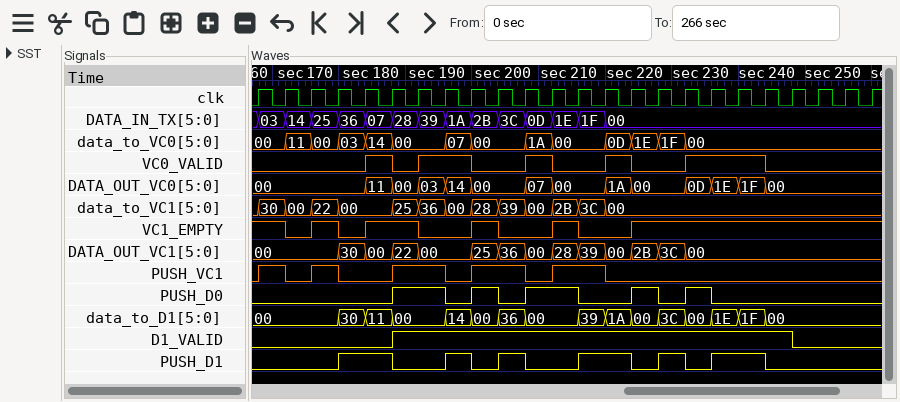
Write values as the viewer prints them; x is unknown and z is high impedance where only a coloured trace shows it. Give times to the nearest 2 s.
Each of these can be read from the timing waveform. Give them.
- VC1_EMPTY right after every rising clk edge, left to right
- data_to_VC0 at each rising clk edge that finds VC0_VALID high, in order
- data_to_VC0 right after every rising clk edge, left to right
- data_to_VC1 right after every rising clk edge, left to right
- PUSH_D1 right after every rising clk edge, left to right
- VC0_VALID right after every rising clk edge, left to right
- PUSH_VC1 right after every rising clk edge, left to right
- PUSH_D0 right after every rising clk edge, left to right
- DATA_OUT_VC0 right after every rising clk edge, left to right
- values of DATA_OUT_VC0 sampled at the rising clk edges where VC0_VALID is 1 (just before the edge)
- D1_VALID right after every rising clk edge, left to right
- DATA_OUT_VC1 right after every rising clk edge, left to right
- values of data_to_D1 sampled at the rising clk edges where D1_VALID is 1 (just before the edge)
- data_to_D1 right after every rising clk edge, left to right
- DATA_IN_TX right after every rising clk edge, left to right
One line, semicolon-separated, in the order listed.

1 0 1 0 1 1 0 0 1 0 0 1 0 0 1 1 1 1 1 1 1 1 1 1; 14, 00, 07, 1A, 0D, 00, 00, 00; 00, 11, 00, 03, 14, 00, 00, 07, 00, 00, 1A, 00, 00, 0D, 1E, 1F, 00, 00, 00, 00, 00, 00, 00, 00; 30, 00, 22, 00, 00, 25, 36, 00, 28, 39, 00, 2B, 3C, 00, 00, 00, 00, 00, 00, 00, 00, 00, 00, 00; 0 0 0 1 1 0 0 1 0 1 0 0 1 1 0 1 0 1 1 0 0 0 0 0; 0 0 0 0 1 0 1 1 0 0 1 0 0 1 0 0 1 1 1 0 0 0 0 0; 1 0 1 0 0 1 1 0 1 1 0 1 1 0 0 0 0 0 0 0 0 0 0 0; 0 0 0 0 0 1 1 0 1 0 1 1 0 0 1 0 1 0 0 0 0 0 0 0; 00, 00, 00, 00, 11, 00, 03, 14, 00, 00, 07, 00, 00, 1A, 00, 00, 0D, 1E, 1F, 00, 00, 00, 00, 00; 11, 03, 14, 07, 1A, 0D, 1E, 1F; 0 0 0 0 0 1 1 1 1 1 1 1 1 1 1 1 1 1 1 1 0 0 0 0; 00, 00, 00, 30, 00, 22, 00, 00, 25, 36, 00, 28, 39, 00, 2B, 3C, 00, 00, 00, 00, 00, 00, 00, 00; 00, 00, 14, 00, 36, 00, 00, 39, 1A, 00, 3C, 00, 1E, 1F, 00; 00, 00, 00, 30, 11, 00, 00, 14, 00, 36, 00, 00, 39, 1A, 00, 3C, 00, 1E, 1F, 00, 00, 00, 00, 00; 03, 14, 25, 36, 07, 28, 39, 1A, 2B, 3C, 0D, 1E, 1F, 00, 00, 00, 00, 00, 00, 00, 00, 00, 00, 00
